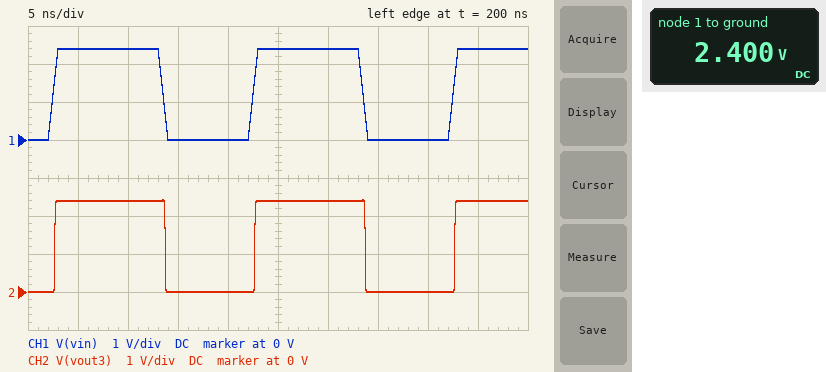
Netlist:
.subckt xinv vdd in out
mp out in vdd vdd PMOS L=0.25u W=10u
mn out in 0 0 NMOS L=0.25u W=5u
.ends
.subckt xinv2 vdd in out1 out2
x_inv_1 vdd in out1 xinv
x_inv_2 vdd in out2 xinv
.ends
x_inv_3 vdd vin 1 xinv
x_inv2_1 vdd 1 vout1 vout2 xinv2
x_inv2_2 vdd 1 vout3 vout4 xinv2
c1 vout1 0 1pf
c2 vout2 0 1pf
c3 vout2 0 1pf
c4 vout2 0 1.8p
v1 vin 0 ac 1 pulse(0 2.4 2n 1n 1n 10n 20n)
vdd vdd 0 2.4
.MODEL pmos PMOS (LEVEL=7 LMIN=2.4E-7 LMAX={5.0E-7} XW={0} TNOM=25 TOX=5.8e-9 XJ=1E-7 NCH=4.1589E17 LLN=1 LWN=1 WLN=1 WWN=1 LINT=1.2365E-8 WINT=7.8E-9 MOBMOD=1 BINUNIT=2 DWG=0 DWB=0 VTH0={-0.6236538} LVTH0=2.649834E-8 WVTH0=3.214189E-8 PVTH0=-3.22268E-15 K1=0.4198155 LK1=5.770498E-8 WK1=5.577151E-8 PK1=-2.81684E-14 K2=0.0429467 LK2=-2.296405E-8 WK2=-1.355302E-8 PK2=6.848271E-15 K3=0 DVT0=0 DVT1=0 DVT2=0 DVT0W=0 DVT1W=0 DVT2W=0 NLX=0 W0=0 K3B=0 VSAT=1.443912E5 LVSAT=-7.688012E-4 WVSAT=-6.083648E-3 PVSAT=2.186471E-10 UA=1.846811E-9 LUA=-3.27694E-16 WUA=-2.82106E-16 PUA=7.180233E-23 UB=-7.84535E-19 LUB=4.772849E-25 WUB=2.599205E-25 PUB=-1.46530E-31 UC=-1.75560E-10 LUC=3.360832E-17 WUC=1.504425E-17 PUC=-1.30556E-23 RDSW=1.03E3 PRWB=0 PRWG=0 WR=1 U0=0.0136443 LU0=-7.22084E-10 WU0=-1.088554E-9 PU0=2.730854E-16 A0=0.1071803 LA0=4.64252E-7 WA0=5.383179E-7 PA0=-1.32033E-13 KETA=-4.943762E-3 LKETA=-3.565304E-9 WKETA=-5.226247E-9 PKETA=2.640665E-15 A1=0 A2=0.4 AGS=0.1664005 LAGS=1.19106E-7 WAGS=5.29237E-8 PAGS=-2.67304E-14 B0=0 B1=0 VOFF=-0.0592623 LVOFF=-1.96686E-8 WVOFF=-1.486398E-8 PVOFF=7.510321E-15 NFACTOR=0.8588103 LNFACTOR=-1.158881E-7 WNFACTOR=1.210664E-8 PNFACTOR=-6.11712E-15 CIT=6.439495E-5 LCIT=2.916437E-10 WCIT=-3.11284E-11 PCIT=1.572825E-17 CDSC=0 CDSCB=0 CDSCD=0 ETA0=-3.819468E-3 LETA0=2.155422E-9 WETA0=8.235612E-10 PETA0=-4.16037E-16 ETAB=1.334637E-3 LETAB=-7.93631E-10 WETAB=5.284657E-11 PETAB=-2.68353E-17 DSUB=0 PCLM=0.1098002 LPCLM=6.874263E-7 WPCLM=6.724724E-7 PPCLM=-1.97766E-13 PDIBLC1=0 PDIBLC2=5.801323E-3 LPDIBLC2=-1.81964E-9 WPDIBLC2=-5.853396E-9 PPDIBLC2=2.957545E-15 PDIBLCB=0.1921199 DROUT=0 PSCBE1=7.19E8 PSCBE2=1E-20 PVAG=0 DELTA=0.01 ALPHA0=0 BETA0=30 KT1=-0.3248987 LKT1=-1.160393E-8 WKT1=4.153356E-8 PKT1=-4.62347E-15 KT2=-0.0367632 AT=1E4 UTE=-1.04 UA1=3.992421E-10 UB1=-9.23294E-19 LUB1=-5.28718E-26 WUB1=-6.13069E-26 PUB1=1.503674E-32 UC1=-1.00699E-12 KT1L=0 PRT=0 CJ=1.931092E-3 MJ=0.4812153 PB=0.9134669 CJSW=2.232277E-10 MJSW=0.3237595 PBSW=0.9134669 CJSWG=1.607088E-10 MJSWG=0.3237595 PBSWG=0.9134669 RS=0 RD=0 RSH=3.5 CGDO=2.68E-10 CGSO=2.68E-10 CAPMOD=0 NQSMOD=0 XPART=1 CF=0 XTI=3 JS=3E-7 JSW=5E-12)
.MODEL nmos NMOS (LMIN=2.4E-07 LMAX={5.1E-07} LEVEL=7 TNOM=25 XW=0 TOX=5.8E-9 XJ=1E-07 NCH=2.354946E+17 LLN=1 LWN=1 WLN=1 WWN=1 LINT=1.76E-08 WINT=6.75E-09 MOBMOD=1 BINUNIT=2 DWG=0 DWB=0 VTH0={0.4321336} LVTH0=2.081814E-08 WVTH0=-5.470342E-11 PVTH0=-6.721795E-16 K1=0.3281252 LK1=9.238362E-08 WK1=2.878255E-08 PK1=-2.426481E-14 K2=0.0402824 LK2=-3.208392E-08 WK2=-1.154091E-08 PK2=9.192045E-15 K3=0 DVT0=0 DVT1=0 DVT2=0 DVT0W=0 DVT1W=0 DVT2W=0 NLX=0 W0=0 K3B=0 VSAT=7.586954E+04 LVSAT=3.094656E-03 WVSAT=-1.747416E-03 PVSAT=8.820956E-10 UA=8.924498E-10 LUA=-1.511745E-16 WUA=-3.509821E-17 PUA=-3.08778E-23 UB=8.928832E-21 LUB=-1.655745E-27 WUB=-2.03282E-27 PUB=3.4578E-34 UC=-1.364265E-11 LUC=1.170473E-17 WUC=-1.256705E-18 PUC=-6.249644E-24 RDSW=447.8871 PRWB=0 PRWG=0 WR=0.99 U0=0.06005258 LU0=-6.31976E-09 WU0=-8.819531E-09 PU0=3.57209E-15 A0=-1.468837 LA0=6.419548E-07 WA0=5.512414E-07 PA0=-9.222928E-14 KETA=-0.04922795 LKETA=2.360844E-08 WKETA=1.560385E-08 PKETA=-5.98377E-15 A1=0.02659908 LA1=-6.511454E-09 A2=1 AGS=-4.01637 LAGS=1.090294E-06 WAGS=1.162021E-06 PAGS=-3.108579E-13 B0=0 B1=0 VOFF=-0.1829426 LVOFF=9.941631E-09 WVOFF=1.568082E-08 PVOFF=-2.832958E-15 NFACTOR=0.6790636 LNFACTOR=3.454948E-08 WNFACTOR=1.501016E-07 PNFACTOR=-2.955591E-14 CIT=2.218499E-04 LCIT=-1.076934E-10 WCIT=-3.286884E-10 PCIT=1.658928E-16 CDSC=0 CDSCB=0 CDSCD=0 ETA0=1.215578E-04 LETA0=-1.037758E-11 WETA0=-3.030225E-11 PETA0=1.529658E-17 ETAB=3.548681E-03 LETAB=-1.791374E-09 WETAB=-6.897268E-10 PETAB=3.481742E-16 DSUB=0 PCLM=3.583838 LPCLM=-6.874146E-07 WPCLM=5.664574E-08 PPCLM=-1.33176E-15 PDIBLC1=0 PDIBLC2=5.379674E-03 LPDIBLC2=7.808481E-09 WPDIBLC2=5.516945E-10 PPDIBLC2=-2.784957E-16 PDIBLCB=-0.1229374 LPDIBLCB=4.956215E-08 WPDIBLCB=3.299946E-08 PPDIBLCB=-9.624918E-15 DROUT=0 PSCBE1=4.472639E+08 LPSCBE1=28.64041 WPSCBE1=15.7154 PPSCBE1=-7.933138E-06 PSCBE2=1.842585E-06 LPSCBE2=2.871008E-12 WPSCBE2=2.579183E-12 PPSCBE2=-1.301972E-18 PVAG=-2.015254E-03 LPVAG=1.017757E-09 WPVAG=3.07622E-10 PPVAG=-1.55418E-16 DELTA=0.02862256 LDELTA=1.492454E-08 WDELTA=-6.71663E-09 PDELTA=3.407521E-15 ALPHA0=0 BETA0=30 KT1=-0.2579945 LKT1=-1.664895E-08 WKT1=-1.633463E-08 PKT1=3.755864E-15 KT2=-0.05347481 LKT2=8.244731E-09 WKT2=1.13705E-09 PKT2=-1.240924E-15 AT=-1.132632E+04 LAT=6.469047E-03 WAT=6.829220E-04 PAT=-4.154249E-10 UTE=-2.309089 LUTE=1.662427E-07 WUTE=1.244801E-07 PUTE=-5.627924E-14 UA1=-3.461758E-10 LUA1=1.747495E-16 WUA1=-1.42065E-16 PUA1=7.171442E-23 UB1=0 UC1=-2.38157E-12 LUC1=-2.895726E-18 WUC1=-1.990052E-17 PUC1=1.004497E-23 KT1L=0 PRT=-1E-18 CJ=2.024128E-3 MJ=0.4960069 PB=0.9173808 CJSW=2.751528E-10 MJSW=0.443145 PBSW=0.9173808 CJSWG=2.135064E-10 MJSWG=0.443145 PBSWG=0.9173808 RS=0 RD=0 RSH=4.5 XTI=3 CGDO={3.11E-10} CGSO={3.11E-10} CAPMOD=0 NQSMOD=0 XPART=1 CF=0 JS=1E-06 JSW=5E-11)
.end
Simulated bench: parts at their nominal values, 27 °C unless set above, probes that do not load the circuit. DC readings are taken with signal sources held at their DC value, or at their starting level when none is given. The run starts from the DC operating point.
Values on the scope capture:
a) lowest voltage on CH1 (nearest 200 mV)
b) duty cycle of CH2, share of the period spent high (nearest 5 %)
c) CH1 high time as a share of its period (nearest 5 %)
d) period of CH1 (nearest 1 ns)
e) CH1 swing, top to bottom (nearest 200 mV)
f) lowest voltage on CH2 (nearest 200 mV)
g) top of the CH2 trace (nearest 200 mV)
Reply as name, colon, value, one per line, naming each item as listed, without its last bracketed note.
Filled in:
lowest voltage on CH1: 0 V
duty cycle of CH2, share of the period spent high: 55 %
CH1 high time as a share of its period: 55 %
period of CH1: 20 ns
CH1 swing, top to bottom: 2.4 V
lowest voltage on CH2: 0 V
top of the CH2 trace: 2.4 V
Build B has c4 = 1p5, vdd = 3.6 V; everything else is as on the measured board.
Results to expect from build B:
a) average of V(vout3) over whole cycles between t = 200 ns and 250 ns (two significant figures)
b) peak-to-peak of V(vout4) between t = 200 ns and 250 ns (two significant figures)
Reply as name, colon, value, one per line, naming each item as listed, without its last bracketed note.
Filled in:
average of V(vout3) over whole cycles between t = 200 ns and 250 ns: 1.9 V
peak-to-peak of V(vout4) between t = 200 ns and 250 ns: 3.6 V
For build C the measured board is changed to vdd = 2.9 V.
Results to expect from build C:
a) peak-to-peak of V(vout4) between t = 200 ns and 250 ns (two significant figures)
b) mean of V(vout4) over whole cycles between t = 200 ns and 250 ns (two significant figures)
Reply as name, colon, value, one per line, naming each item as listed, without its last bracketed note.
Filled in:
peak-to-peak of V(vout4) between t = 200 ns and 250 ns: 2.9 V
mean of V(vout4) over whole cycles between t = 200 ns and 250 ns: 1.6 V
